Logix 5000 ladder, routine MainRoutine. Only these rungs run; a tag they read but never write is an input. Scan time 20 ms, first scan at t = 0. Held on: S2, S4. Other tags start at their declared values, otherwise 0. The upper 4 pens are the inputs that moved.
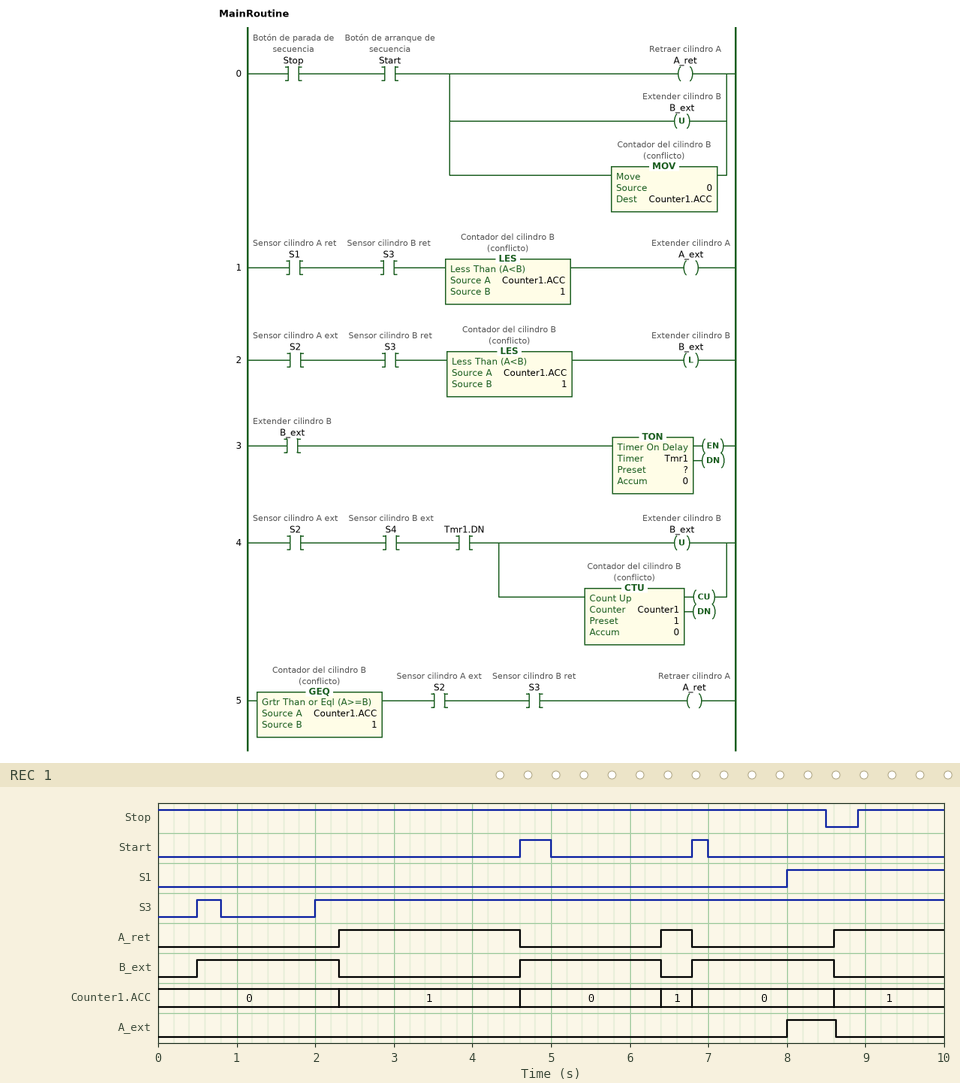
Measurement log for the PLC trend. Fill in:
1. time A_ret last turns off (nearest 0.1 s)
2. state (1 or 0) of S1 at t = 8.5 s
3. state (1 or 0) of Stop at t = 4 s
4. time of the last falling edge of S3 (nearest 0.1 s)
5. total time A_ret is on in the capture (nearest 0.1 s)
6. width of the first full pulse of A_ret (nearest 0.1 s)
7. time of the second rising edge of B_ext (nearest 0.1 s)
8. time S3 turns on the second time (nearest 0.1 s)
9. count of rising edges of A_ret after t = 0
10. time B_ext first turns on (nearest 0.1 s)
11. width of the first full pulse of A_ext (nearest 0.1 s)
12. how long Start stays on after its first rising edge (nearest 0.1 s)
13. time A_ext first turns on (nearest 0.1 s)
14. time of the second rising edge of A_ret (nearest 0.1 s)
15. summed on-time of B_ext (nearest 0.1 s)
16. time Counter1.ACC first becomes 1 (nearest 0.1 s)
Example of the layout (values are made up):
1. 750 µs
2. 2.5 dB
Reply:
1. 6.8 s
2. 1
3. 1
4. 0.8 s
5. 4.1 s
6. 2.3 s
7. 4.6 s
8. 2.0 s
9. 3
10. 0.5 s
11. 0.6 s
12. 0.4 s
13. 8.0 s
14. 6.4 s
15. 5.4 s
16. 2.3 s
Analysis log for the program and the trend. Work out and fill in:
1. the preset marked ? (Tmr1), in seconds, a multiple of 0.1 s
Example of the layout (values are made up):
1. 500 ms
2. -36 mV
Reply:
1. 1.8 s
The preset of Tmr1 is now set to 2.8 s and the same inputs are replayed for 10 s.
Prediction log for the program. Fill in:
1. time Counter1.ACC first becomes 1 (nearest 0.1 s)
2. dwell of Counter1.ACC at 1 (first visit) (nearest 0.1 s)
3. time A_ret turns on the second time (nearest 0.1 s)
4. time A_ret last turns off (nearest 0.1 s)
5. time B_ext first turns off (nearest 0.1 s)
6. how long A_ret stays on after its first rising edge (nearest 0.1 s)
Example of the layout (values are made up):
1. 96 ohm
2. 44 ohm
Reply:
1. 3.3 s
2. 1.3 s
3. 7.4 s
4. 4.6 s
5. 3.3 s
6. 1.3 s
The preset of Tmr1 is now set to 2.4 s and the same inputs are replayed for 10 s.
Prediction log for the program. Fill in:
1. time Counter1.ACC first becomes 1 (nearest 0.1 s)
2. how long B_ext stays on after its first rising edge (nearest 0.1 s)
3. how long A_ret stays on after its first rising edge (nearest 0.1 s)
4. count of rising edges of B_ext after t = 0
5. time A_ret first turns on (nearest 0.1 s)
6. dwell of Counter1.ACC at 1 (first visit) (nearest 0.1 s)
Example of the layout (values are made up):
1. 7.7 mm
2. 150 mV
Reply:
1. 2.9 s
2. 2.4 s
3. 1.7 s
4. 2
5. 2.9 s
6. 1.7 s
